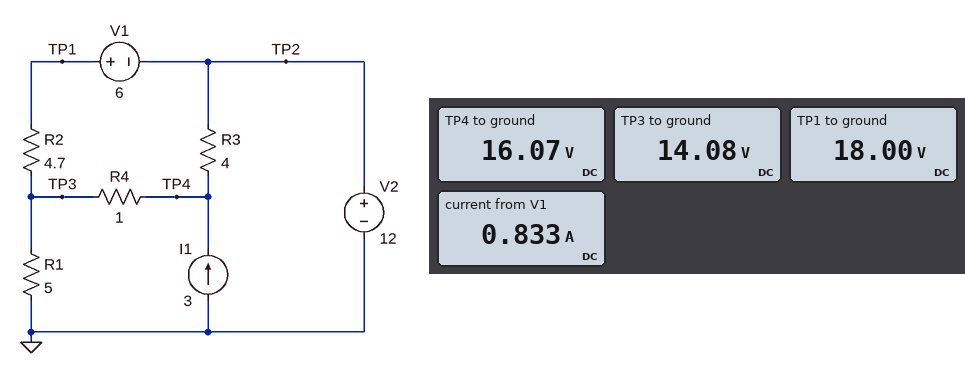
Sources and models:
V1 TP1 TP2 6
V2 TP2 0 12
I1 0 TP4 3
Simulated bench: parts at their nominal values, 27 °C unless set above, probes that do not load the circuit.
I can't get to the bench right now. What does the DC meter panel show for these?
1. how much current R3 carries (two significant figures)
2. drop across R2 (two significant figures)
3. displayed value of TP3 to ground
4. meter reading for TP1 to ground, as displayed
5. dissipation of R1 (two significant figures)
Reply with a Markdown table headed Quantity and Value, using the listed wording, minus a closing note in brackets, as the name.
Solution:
| Quantity | Value |
|---|---|
| how much current R3 carries | 1.0 A |
| drop across R2 | 3.9 V |
| displayed value of TP3 to ground | 14.08 V |
| meter reading for TP1 to ground, as displayed | 18.00 V |
| dissipation of R1 | 40 W |
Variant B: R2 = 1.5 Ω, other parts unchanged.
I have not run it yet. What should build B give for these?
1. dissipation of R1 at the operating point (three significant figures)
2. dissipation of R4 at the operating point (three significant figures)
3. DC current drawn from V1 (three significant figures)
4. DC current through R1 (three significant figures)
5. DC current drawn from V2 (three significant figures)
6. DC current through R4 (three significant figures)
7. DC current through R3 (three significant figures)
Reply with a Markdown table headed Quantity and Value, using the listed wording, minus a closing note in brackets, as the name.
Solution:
| Quantity | Value |
|---|---|
| dissipation of R1 at the operating point | 49.6 W |
| dissipation of R4 at the operating point | 2.72 W |
| DC current drawn from V1 | 1.50 A |
| DC current through R1 | 3.15 A |
| DC current drawn from V2 | 150 mA |
| DC current through R4 | 1.65 A |
| DC current through R3 | 1.35 A |
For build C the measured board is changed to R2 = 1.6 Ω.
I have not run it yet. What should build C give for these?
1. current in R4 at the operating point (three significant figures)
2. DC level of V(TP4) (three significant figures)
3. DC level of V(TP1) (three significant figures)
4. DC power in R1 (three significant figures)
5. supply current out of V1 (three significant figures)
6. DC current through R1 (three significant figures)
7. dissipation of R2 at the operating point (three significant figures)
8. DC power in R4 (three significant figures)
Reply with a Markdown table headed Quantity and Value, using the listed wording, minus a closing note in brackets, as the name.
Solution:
| Quantity | Value |
|---|---|
| current in R4 at the operating point | 1.67 A |
| DC level of V(TP4) | 17.3 V |
| DC level of V(TP1) | 18.0 V |
| DC power in R1 | 49.0 W |
| supply current out of V1 | 1.46 A |
| DC current through R1 | 3.13 A |
| dissipation of R2 at the operating point | 3.43 W |
| DC power in R4 | 2.78 W |
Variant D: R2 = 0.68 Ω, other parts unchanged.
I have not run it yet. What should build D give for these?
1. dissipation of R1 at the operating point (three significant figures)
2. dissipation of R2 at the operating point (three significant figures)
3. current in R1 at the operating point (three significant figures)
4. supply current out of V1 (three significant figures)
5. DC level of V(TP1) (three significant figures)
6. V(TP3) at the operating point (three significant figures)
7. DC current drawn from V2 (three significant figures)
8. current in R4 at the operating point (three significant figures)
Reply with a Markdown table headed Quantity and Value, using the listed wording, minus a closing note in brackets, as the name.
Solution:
| Quantity | Value |
|---|---|
| dissipation of R1 at the operating point | 55.9 W |
| dissipation of R2 at the operating point | 2.42 W |
| current in R1 at the operating point | 3.34 A |
| supply current out of V1 | 1.89 A |
| DC level of V(TP1) | 18.0 V |
| V(TP3) at the operating point | 16.7 V |
| DC current drawn from V2 | 343 mA |
| current in R4 at the operating point | 1.46 A |
